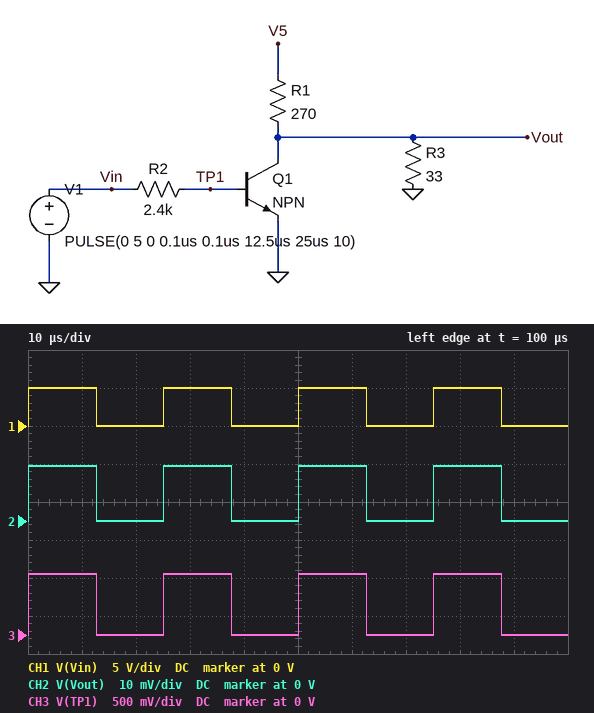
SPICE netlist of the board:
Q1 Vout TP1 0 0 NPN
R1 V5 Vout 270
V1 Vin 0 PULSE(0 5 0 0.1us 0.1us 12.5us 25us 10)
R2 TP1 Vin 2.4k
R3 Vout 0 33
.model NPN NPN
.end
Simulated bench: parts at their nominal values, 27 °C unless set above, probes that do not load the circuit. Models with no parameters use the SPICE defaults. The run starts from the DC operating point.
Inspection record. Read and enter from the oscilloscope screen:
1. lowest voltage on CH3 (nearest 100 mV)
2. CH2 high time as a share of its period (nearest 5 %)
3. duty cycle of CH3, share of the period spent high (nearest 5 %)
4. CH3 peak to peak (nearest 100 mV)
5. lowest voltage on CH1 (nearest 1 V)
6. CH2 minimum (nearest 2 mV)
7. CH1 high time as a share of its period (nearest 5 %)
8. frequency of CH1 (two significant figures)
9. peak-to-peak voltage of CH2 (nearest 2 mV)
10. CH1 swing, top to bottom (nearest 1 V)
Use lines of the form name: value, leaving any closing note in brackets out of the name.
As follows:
lowest voltage on CH3: 0 V
CH2 high time as a share of its period: 50 %
duty cycle of CH3, share of the period spent high: 50 %
CH3 peak to peak: 800 mV
lowest voltage on CH1: 0 V
CH2 minimum: 0 V
CH1 high time as a share of its period: 50 %
frequency of CH1: 40 kHz
peak-to-peak voltage of CH2: 14 mV
CH1 swing, top to bottom: 5 V
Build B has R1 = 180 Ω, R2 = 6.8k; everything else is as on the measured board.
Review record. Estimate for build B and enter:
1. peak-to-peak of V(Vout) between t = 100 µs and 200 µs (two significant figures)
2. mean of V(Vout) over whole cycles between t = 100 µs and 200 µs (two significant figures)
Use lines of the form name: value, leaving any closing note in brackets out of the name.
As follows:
peak-to-peak of V(Vout) between t = 100 µs and 200 µs: 10 mV
mean of V(Vout) over whole cycles between t = 100 µs and 200 µs: 5.2 mV
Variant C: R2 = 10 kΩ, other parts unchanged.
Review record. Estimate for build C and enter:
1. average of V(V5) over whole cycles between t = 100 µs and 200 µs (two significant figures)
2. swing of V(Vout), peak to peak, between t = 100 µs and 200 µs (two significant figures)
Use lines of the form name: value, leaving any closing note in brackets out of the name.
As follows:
average of V(V5) over whole cycles between t = 100 µs and 200 µs: 4.3 mV
swing of V(Vout), peak to peak, between t = 100 µs and 200 µs: 8.5 mV
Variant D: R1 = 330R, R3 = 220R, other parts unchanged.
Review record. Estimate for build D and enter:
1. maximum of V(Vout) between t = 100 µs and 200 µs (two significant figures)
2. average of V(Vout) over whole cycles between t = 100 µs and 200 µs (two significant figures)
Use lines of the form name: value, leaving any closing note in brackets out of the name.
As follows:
maximum of V(Vout) between t = 100 µs and 200 µs: 17 mV
average of V(Vout) over whole cycles between t = 100 µs and 200 µs: 8.8 mV
